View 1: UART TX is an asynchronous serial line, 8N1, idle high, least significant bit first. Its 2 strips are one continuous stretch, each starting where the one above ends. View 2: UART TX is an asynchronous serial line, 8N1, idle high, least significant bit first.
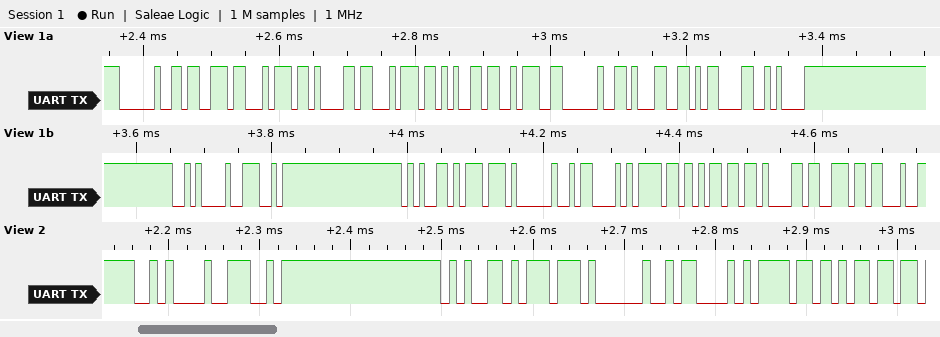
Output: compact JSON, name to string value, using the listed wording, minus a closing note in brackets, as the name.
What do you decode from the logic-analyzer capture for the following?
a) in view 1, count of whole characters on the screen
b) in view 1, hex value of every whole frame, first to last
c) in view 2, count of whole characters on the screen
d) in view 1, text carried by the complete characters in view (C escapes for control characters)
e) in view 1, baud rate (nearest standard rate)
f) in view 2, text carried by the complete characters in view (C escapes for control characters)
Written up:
{"in view 1, count of whole characters on the screen": "21", "in view 1, hex value of every whole frame, first to last": "20 73 74 61 74 65 3A 20 31 0D 0A 0A 4E 65 77 20 43 6F 6D 61 6E", "in view 2, count of whole characters on the screen": "8", "in view 1, text carried by the complete characters in view": "\" state: 1\\r\\n\\nNew Coman\"", "in view 1, baud rate": "115200 baud", "in view 2, text carried by the complete characters in view": "\"\\nNew Com\""}
